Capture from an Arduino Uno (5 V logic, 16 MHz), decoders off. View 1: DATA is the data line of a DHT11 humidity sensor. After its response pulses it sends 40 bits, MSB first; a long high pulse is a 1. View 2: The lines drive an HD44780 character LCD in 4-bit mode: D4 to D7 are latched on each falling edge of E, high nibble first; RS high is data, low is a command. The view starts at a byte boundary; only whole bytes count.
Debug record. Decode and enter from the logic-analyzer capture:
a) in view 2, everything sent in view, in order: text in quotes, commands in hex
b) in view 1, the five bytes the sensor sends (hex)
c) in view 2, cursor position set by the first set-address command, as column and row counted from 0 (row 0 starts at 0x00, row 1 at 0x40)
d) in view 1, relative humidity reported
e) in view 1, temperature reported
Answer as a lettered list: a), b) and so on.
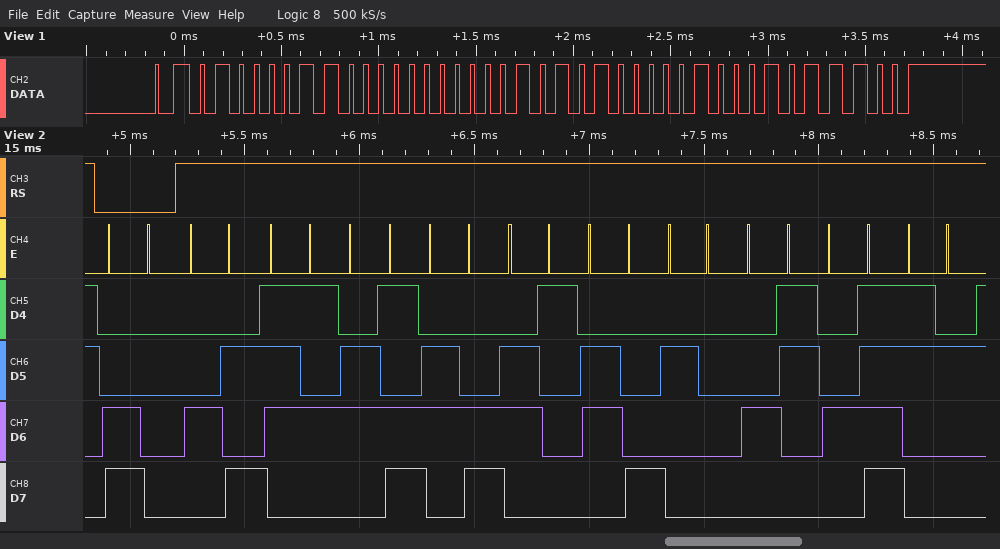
a) 0xC0 "Jumlah CO2"
b) 43 00 15 04 5C
c) column 0, row 1
d) 67 %
e) 21.4 °C
